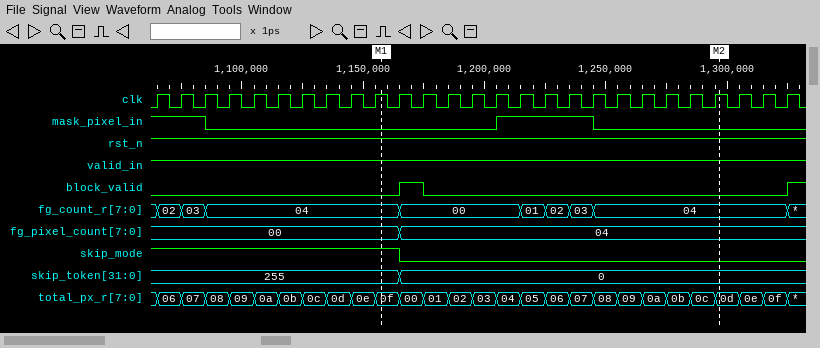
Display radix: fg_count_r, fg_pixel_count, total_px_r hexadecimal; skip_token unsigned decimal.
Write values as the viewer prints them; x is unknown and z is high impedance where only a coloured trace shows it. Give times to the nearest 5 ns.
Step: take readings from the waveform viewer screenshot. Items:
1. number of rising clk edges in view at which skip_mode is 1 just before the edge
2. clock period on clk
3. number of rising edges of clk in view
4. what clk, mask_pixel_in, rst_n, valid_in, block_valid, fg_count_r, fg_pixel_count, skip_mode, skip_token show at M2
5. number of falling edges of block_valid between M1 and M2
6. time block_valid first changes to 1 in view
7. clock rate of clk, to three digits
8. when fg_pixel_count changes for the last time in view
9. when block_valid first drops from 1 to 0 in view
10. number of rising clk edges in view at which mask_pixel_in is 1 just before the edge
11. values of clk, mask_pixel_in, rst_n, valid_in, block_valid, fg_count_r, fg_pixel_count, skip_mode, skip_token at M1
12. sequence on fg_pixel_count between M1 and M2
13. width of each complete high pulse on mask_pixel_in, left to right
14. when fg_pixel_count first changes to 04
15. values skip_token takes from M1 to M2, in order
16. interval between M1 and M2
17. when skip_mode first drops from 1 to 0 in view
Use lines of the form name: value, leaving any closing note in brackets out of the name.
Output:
number of rising clk edges in view at which skip_mode is 1 just before the edge: 11
clock period on clk: 10 ns
number of rising edges of clk in view: 27
what clk, mask_pixel_in, rst_n, valid_in, block_valid, fg_count_r, fg_pixel_count, skip_mode, skip_token show at M2: clk=1, mask_pixel_in=0, rst_n=1, valid_in=1, block_valid=0, fg_count_r=04, fg_pixel_count=04, skip_mode=0, skip_token=0
number of falling edges of block_valid between M1 and M2: 1
time block_valid first changes to 1 in view: 1165 ns
clock rate of clk, to three digits: 100 MHz
when fg_pixel_count changes for the last time in view: 1165 ns
when block_valid first drops from 1 to 0 in view: 1175 ns
number of rising clk edges in view at which mask_pixel_in is 1 just before the edge: 7
values of clk, mask_pixel_in, rst_n, valid_in, block_valid, fg_count_r, fg_pixel_count, skip_mode, skip_token at M1: clk=1, mask_pixel_in=0, rst_n=1, valid_in=1, block_valid=0, fg_count_r=04, fg_pixel_count=00, skip_mode=1, skip_token=255
sequence on fg_pixel_count between M1 and M2: 00, 04
width of each complete high pulse on mask_pixel_in, left to right: 40 ns
when fg_pixel_count first changes to 04: 1165 ns
values skip_token takes from M1 to M2, in order: 255, 0
interval between M1 and M2: 140 ns
when skip_mode first drops from 1 to 0 in view: 1165 ns
